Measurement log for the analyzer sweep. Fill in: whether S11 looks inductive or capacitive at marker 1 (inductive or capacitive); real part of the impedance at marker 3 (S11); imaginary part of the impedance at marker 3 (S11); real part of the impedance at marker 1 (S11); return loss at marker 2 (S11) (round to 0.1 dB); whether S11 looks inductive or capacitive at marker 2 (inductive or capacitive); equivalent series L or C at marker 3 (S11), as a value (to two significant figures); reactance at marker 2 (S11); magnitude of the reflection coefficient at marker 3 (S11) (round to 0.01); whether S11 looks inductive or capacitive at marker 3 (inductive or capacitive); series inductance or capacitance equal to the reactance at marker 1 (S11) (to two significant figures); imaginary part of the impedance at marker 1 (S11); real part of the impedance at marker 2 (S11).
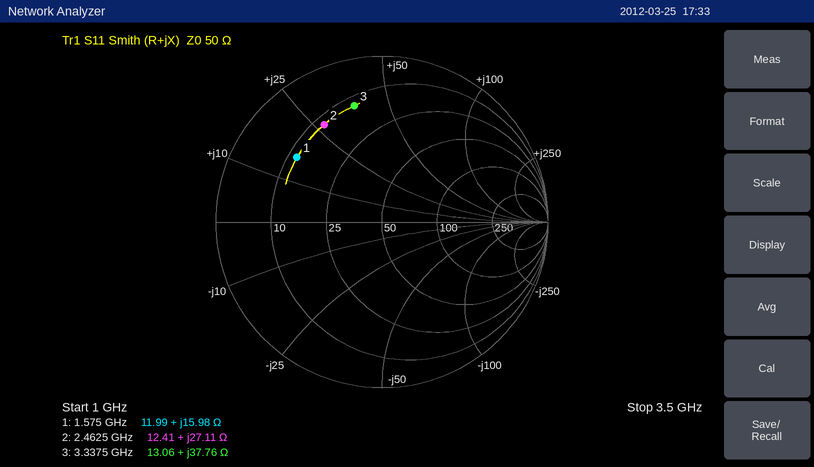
inductive
13.06 Ω
+37.76 Ω
11.99 Ω
3.3 dB
inductive
1.8 nH
+27.11 Ω
0.72
inductive
1.6 nH
+15.98 Ω
12.41 Ω
